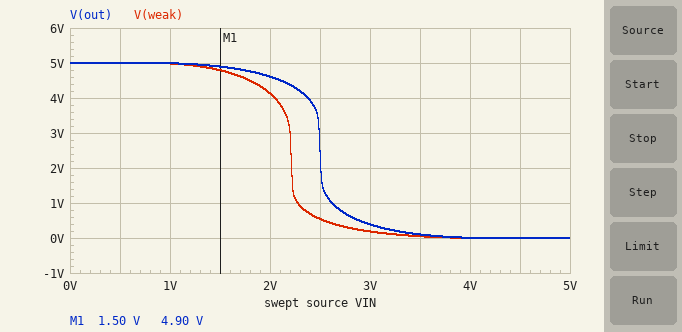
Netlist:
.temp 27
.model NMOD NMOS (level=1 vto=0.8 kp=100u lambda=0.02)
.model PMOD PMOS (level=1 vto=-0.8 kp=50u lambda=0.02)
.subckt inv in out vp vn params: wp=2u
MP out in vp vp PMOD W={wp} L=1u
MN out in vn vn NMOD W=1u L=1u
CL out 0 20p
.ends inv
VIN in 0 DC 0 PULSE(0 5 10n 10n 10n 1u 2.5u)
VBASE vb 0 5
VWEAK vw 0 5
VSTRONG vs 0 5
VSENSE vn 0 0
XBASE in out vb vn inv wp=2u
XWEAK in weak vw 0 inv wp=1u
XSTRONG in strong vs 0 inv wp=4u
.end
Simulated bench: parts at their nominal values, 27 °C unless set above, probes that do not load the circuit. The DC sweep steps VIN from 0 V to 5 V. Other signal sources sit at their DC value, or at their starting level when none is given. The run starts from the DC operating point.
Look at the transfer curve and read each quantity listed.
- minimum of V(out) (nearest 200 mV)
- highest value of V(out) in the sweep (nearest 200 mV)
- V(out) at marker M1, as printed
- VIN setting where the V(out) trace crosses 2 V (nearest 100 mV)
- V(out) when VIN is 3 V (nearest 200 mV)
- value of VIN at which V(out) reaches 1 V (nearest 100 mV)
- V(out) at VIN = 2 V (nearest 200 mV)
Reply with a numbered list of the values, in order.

1. 0 V
2. 5.0 V
3. 4.90 V
4. 2.5 V
5. 400 mV
6. 2.6 V
7. 4.6 V
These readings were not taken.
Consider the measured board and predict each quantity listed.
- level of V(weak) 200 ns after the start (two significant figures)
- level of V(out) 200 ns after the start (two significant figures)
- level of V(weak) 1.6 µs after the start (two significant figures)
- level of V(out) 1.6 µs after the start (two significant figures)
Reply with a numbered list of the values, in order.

1. 220 mV
2. 220 mV
3. 5.0 V
4. 5.0 V
